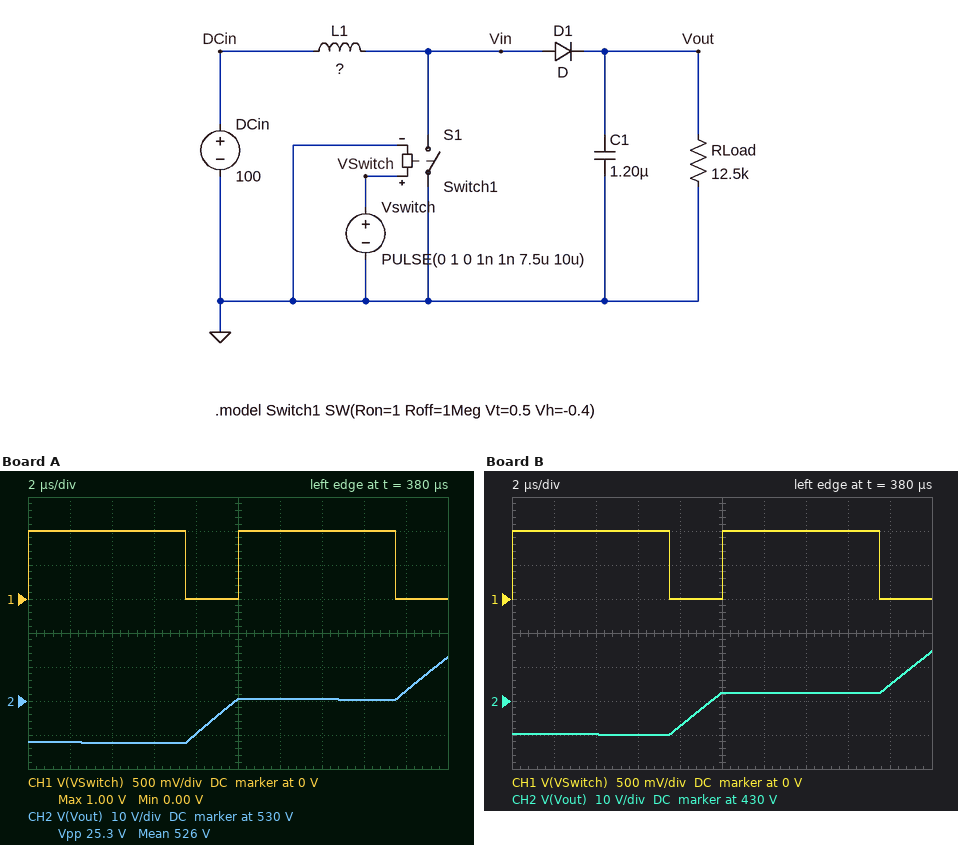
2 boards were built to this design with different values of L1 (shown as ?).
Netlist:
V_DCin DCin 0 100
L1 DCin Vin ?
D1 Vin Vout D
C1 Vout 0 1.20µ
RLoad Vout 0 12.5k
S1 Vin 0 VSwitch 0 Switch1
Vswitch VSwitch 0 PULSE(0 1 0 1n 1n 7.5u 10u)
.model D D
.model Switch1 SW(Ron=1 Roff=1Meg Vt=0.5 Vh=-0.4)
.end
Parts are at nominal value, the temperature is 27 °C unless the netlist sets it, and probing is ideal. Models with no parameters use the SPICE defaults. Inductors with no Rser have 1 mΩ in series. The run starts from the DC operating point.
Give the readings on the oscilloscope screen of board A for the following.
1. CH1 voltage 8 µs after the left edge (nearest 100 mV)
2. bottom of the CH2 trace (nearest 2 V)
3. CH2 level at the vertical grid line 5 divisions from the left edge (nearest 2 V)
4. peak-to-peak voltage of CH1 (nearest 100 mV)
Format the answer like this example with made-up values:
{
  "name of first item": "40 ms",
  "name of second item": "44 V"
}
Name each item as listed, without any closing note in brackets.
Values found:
{
  "CH1 voltage 8 µs after the left edge": "0 V",
  "bottom of the CH2 trace": "518 V",
  "CH2 level at the vertical grid line 5 divisions from the left edge": "530 V",
  "peak-to-peak voltage of CH1": "1.0 V"
}
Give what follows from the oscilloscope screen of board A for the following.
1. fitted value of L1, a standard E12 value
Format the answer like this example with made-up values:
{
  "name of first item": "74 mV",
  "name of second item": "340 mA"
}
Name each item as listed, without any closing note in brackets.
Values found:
{
  "fitted value of L1, a standard E12 value": "1.8 mH"
}
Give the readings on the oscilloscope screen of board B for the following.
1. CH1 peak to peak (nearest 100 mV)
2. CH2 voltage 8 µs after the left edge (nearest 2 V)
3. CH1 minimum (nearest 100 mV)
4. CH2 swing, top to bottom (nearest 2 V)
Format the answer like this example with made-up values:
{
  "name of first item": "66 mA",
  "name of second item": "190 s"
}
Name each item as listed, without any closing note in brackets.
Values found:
{
  "CH1 peak to peak": "1.0 V",
  "CH2 voltage 8 µs after the left edge": "422 V",
  "CH1 minimum": "0 V",
  "CH2 swing, top to bottom": "24 V"
}
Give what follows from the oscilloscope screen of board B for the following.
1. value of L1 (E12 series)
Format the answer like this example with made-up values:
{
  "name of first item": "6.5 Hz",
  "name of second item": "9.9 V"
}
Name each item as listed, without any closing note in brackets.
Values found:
{
  "value of L1": "2.7 mH"
}
